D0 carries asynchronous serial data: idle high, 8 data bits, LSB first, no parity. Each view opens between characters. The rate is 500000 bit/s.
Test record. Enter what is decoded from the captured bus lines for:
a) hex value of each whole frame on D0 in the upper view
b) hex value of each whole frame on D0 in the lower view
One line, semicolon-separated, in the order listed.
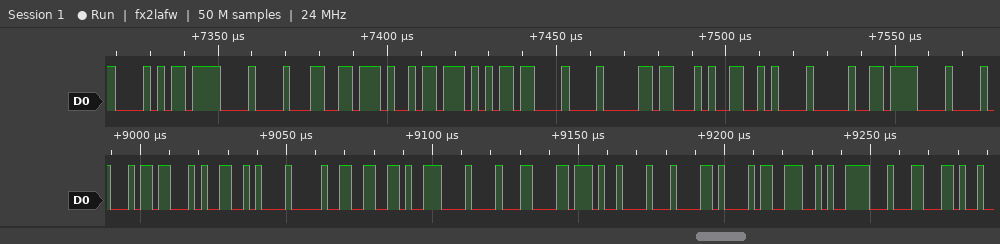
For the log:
A8, 0F, 88, 76, DA, B5, 08, B0, 94, 0A, 90, 0F; B4, 94, 0A, 90, 66, 0E, 88, D8, 09, 84, A1, 4E, 1E, 8C
